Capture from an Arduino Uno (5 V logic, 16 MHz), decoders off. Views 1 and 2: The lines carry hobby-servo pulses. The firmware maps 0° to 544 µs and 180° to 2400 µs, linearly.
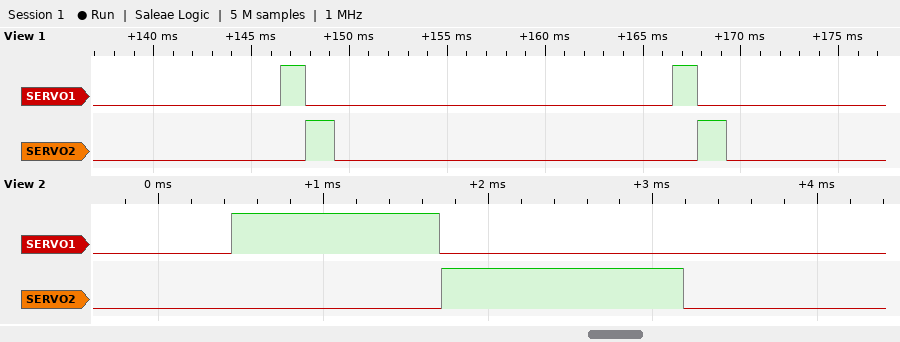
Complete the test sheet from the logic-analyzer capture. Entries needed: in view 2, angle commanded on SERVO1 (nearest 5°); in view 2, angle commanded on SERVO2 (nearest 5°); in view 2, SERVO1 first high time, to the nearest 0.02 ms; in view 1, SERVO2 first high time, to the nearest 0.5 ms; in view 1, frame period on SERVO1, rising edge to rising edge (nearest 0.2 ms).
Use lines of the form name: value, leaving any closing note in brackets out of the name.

in view 2, angle commanded on SERVO1: 70°
in view 2, angle commanded on SERVO2: 90°
in view 2, SERVO1 first high time, to the nearest 0.02 ms: 1.26 ms
in view 1, SERVO2 first high time, to the nearest 0.5 ms: 1.5 ms
in view 1, frame period on SERVO1, rising edge to rising edge: 20.0 ms
